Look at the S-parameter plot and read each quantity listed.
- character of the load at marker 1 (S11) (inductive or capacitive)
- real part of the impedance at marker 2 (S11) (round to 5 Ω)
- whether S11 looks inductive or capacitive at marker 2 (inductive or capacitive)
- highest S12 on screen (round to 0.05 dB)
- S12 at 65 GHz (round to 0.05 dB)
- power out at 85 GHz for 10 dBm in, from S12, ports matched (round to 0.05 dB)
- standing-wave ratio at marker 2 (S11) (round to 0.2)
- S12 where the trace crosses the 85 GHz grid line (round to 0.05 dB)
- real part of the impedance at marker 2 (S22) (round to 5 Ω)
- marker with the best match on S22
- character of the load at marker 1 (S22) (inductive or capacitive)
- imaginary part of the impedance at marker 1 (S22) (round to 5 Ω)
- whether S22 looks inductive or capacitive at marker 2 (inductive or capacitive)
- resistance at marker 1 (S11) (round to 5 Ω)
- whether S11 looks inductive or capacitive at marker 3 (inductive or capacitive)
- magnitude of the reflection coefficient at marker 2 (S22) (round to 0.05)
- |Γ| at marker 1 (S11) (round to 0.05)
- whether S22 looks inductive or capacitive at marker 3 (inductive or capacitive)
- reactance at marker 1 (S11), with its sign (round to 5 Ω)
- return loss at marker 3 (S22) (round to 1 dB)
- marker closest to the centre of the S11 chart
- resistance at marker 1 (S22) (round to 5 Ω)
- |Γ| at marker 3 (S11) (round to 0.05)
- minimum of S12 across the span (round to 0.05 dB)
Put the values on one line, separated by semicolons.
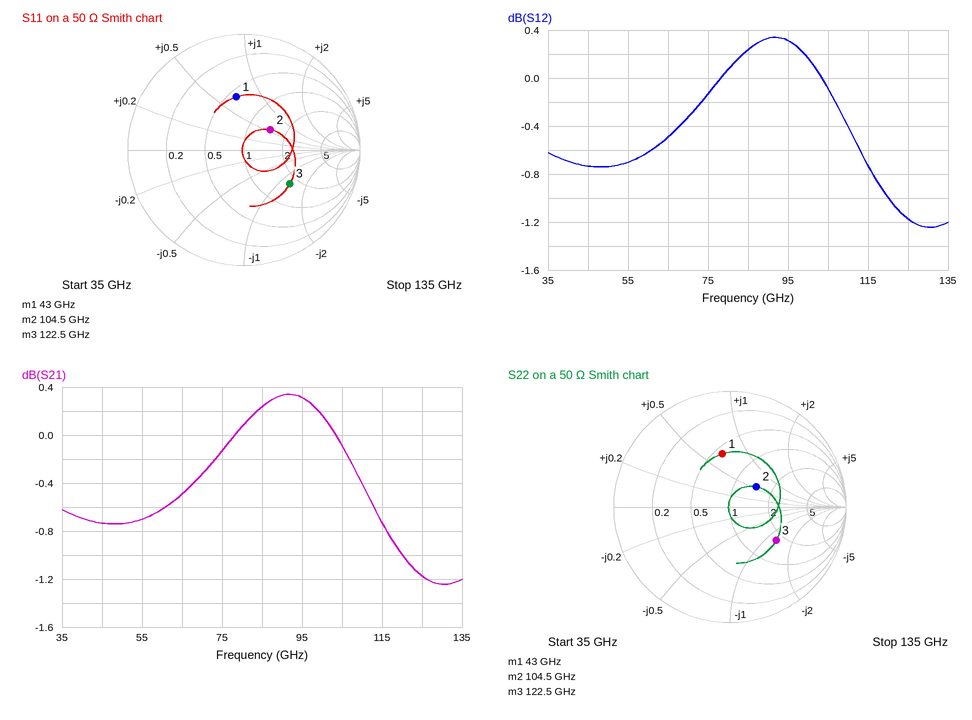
inductive; 75 Ω; inductive; 0.35 dB; -0.50 dB; 10.25 dBm; 1.8; 0.25 dB; 75 Ω; marker 2; inductive; +35 Ω; inductive; 30 Ω; capacitive; 0.30; 0.45; capacitive; +35 Ω; 6 dB; marker 2; 30 Ω; 0.50; -1.25 dB
